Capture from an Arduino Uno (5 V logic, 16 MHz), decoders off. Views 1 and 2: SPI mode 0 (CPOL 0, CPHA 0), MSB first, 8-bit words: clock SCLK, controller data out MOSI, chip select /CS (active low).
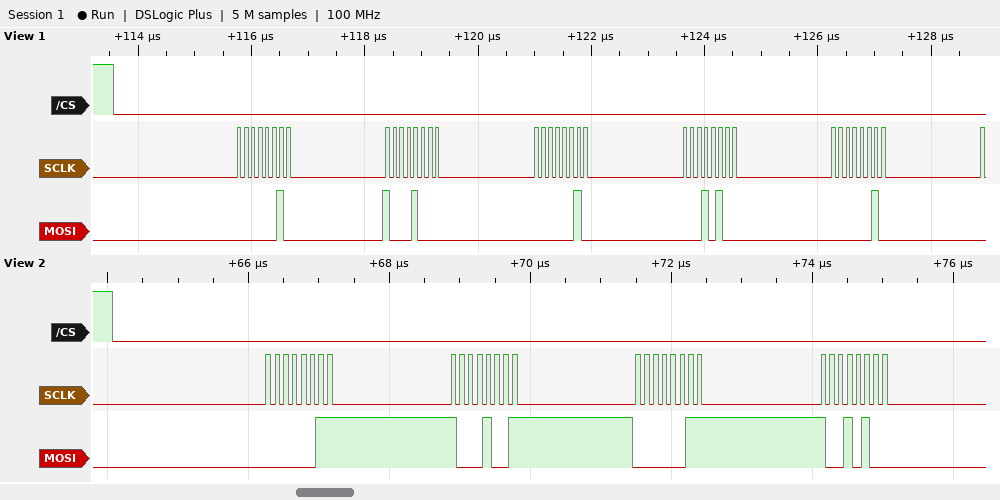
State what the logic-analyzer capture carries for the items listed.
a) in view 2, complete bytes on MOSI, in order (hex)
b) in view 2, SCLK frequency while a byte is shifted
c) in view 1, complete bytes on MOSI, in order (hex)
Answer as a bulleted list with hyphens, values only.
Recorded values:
- 03 89 03 94
- 8 MHz
- 02 88 02 14 02
